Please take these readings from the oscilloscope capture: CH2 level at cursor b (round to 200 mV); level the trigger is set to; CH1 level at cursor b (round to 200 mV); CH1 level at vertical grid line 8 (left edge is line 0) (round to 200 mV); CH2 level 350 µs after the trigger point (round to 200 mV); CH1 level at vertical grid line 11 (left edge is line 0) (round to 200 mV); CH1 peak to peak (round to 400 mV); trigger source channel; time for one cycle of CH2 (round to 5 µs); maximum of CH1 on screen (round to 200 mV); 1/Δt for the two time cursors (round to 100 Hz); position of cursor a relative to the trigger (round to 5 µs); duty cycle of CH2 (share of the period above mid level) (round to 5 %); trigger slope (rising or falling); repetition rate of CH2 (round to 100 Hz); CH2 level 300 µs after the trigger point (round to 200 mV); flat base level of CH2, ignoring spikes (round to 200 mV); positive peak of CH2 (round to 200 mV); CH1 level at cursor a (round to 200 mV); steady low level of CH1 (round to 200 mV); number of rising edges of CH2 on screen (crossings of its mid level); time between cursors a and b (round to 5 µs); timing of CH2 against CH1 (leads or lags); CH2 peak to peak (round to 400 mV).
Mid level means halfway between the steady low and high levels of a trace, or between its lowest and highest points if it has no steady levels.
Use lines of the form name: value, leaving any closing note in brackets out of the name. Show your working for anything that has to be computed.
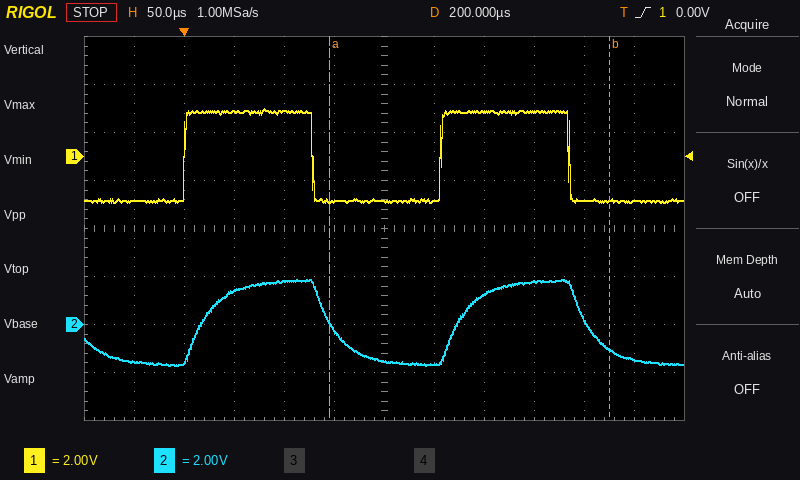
CH2 level at cursor b: -1.0 V
level the trigger is set to: 0.00 V
CH1 level at cursor b: -1.8 V
CH1 level at vertical grid line 8 (left edge is line 0): 1.8 V
CH2 level 350 µs after the trigger point: 1.8 V
CH1 level at vertical grid line 11 (left edge is line 0): -1.8 V
CH1 peak to peak: 4.0 V
trigger source channel: CH1
time for one cycle of CH2: 255 µs
maximum of CH1 on screen: 2.0 V
1/Δt for the two time cursors: 1 / 280 µs ≈ 3.6 kHz
position of cursor a relative to the trigger: +145 µs
duty cycle of CH2 (share of the period above mid level): 50 %
trigger slope: rising
repetition rate of CH2: 1 / 255 µs ≈ 3.9 kHz
CH2 level 300 µs after the trigger point: 1.2 V
flat base level of CH2, ignoring spikes: -1.6 V
positive peak of CH2: 1.8 V
CH1 level at cursor a: -1.8 V
steady low level of CH1: -1.8 V
number of rising edges of CH2 on screen: 2
time between cursors a and b: 280 µs
timing of CH2 against CH1: lags
CH2 peak to peak: 3.6 V
